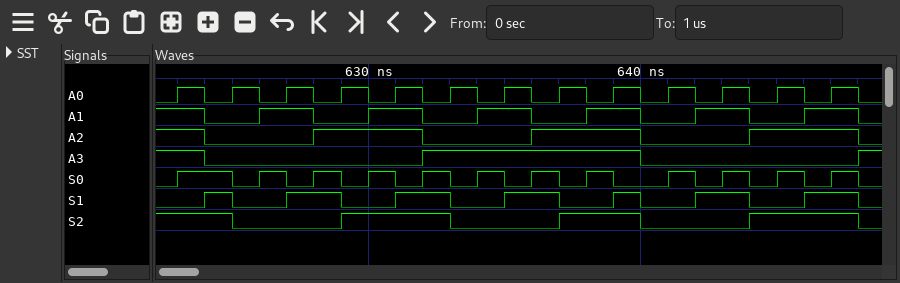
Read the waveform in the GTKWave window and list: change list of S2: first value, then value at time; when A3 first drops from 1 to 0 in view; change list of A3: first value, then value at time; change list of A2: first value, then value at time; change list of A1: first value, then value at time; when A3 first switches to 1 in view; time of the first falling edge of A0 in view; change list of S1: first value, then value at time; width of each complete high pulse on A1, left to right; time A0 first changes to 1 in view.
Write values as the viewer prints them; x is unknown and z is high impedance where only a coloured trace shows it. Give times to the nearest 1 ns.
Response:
1, 0 at 625 ns, 1 at 629 ns, 0 at 633 ns, 1 at 637 ns, 0 at 640 ns, 1 at 644 ns, 0 at 648 ns
624 ns
1, 0 at 624 ns, 1 at 632 ns, 0 at 640 ns, 1 at 648 ns
1, 0 at 624 ns, 1 at 628 ns, 0 at 632 ns, 1 at 636 ns, 0 at 640 ns, 1 at 644 ns, 0 at 648 ns
1, 0 at 624 ns, 1 at 626 ns, 0 at 628 ns, 1 at 630 ns, 0 at 632 ns, 1 at 634 ns, 0 at 636 ns, 1 at 638 ns, 0 at 640 ns, 1 at 642 ns, 0 at 644 ns, 1 at 646 ns, 0 at 648 ns
632 ns
624 ns
0, 1 at 624 ns, 0 at 625 ns, 1 at 627 ns, 0 at 629 ns, 1 at 631 ns, 0 at 633 ns, 1 at 635 ns, 0 at 637 ns, 1 at 639 ns, 0 at 640 ns, 1 at 642 ns, 0 at 644 ns, 1 at 646 ns, 0 at 648 ns
2 ns, 2 ns, 2 ns, 2 ns, 2 ns, 2 ns
623 ns
